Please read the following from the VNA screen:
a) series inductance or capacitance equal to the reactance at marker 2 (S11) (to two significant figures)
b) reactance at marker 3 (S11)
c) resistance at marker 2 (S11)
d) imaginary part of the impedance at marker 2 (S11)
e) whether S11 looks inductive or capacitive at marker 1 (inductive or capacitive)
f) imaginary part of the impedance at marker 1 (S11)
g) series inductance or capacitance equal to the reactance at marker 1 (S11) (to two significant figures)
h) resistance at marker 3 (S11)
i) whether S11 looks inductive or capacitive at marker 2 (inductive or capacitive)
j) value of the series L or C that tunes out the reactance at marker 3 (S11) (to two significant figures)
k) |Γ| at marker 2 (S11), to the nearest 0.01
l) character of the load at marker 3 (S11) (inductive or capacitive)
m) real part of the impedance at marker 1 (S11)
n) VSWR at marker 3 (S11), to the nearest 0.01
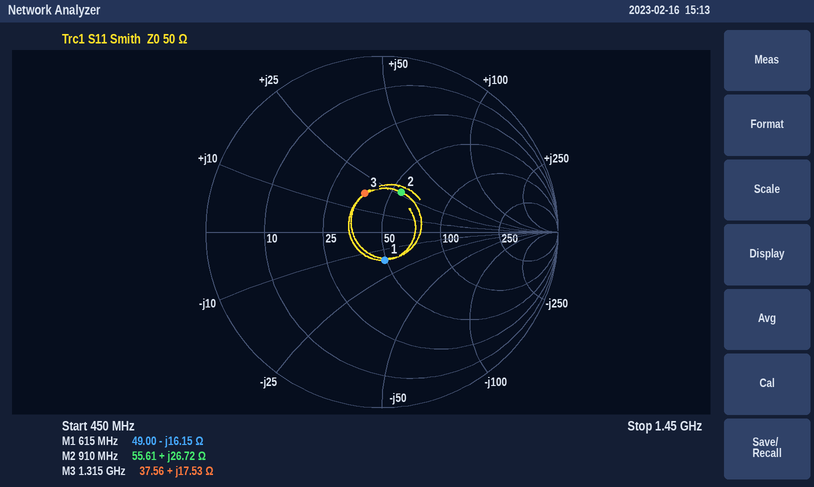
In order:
4.7 nH
+17.53 Ω
55.61 Ω
+26.72 Ω
capacitive
-16.15 Ω
16 pF
37.56 Ω
inductive
6.9 pF
0.25
inductive
49.00 Ω
1.63
